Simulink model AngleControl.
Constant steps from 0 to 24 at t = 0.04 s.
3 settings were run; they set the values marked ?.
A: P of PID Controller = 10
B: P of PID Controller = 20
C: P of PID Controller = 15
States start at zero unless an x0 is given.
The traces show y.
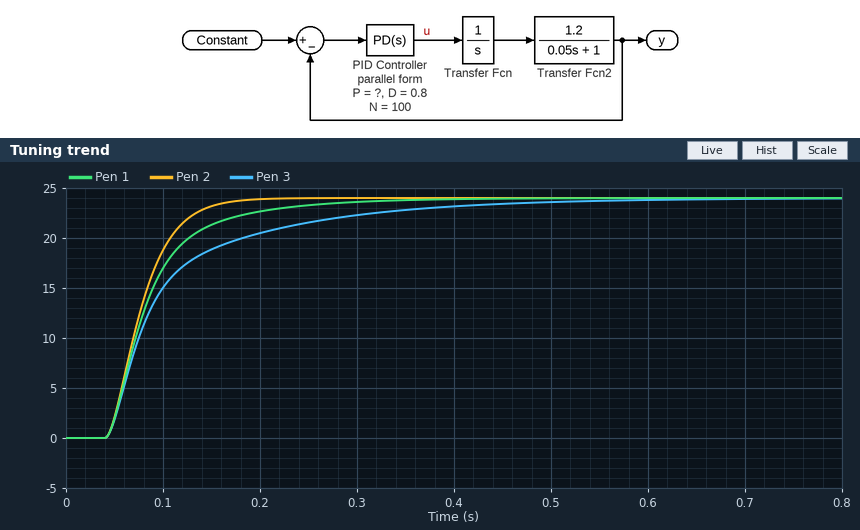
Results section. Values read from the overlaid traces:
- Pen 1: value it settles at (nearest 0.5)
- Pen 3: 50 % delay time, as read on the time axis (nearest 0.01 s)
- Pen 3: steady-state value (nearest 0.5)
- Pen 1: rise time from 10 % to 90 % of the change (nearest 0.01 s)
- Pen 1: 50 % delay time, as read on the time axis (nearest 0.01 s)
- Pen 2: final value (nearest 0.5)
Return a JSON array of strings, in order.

["24.0", "0.08 s", "24.0", "0.11 s", "0.08 s", "24.0"]
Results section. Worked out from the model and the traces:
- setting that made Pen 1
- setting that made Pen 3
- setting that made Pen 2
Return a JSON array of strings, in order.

["C", "A", "B"]
